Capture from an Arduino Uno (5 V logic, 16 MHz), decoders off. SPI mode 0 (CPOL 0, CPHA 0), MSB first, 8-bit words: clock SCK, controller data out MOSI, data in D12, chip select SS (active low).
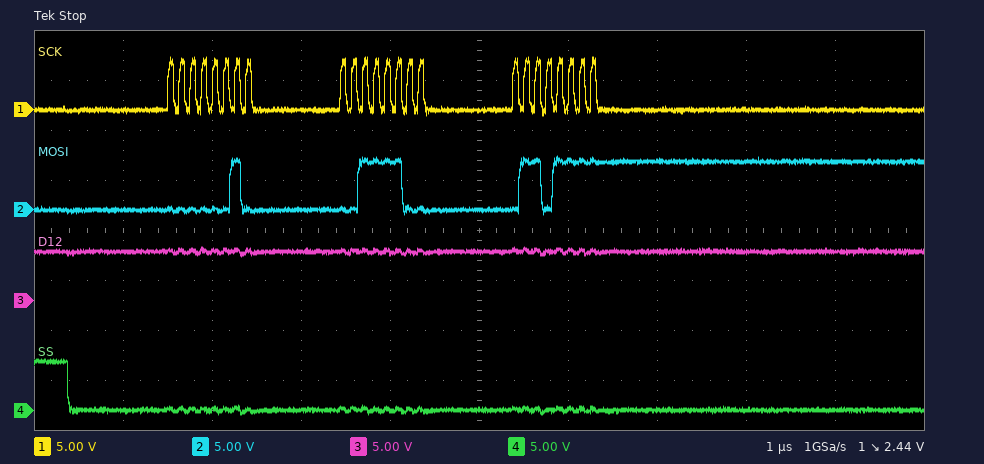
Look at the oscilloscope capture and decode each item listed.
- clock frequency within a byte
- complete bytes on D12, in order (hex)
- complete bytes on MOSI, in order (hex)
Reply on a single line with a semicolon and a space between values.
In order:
8 MHz; FF FF FF; 02 3C 6F
